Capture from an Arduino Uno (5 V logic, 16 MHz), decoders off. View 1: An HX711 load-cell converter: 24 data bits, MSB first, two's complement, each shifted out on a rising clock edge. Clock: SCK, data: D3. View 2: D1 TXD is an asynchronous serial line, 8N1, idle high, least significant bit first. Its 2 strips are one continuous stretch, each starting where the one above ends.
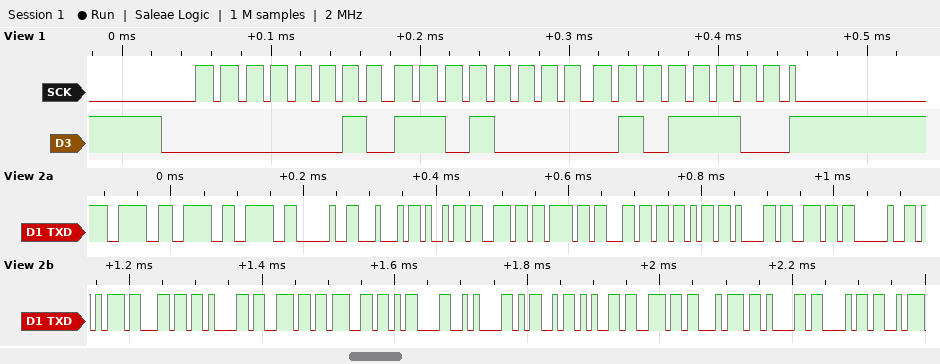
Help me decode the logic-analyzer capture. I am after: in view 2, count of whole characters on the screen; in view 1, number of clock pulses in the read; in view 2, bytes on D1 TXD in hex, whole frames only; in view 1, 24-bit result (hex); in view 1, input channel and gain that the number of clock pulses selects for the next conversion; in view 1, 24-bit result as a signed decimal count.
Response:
26
25
3E 3E 3E 20 44 69 6E 6F 6C 6B 61 6E 20 75 6C 61 6E 67 0D 0A 4D 65 6E 74 61 68
0x02D05C
channel A, gain 128
184412
